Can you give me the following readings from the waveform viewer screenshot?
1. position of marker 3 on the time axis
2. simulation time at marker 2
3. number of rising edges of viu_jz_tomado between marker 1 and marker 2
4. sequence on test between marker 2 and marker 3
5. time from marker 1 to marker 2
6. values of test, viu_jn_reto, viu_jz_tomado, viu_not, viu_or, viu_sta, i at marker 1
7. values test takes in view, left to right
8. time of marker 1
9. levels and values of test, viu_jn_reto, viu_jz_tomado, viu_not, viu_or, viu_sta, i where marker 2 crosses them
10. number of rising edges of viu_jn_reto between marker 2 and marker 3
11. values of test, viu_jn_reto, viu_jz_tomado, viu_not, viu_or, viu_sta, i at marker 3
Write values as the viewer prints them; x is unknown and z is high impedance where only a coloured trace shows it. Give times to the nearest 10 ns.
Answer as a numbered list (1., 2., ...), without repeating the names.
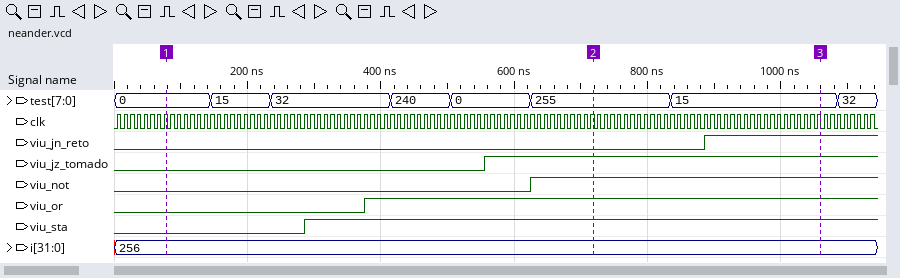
1. 1060 ns
2. 720 ns
3. 1
4. 255, 15
5. 640 ns
6. test=0, viu_jn_reto=0, viu_jz_tomado=0, viu_not=0, viu_or=0, viu_sta=0, i=256
7. 0, 15, 32, 240, 0, 255, 15, 32
8. 80 ns
9. test=255, viu_jn_reto=0, viu_jz_tomado=1, viu_not=1, viu_or=1, viu_sta=1, i=256
10. 1
11. test=15, viu_jn_reto=1, viu_jz_tomado=1, viu_not=1, viu_or=1, viu_sta=1, i=256
